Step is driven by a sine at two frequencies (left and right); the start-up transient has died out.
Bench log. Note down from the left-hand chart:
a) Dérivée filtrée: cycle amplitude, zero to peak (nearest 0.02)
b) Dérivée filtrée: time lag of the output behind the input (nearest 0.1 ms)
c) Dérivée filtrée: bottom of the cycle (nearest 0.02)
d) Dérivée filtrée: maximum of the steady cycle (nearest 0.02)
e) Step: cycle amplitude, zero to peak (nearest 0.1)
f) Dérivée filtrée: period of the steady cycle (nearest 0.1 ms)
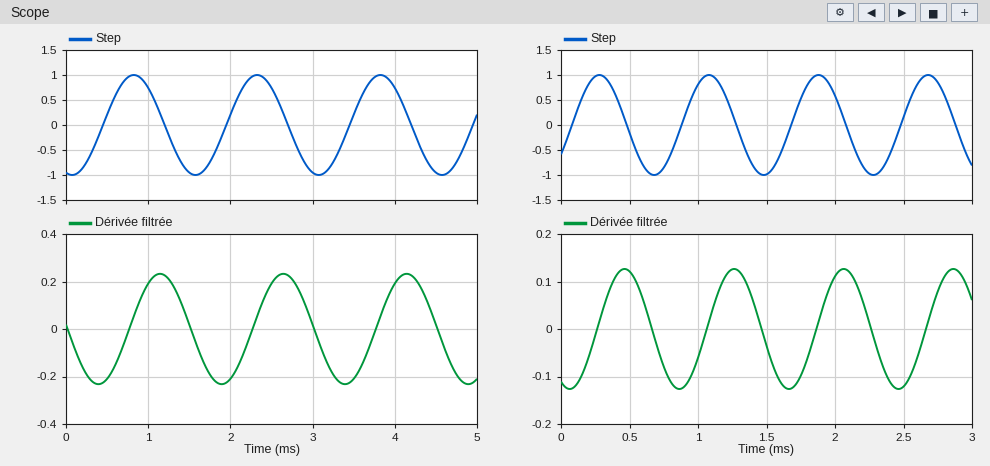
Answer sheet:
0.24
0.3 ms
-0.24
0.24
1.0
1.5 ms
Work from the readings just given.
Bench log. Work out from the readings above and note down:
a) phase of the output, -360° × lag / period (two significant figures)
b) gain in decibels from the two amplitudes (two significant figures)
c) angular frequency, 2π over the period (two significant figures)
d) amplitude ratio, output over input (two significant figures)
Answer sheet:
-72°
-12 dB
4.2 rad/ms
0.24
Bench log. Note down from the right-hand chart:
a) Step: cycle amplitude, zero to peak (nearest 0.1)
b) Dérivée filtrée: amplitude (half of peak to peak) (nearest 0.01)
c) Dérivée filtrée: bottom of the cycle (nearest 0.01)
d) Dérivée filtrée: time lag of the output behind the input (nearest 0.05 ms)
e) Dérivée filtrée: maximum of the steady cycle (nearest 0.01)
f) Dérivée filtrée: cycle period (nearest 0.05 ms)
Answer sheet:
1.0
0.13
-0.13
0.20 ms
0.13
0.80 ms
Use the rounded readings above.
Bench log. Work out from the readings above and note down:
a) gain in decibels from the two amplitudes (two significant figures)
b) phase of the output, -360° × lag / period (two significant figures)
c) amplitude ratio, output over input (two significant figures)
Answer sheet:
-18 dB
-90°
0.13
